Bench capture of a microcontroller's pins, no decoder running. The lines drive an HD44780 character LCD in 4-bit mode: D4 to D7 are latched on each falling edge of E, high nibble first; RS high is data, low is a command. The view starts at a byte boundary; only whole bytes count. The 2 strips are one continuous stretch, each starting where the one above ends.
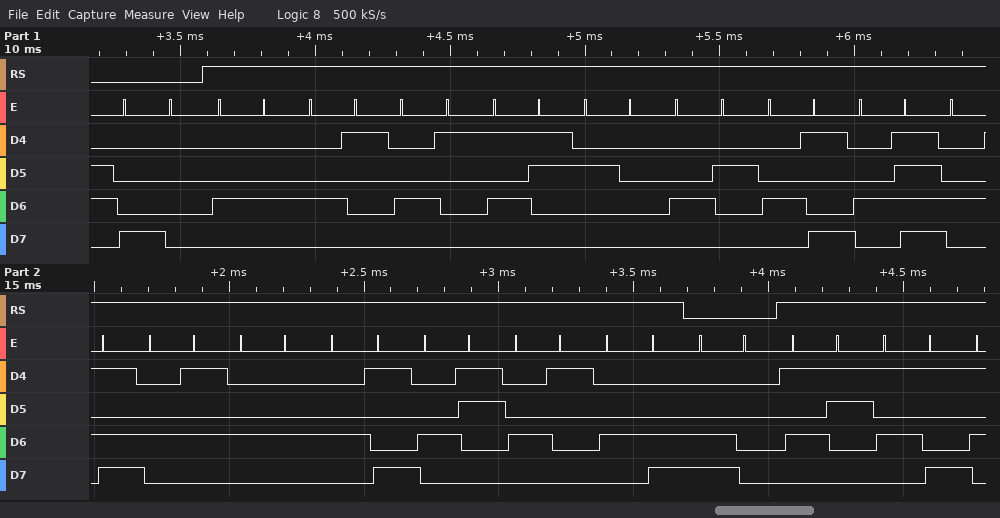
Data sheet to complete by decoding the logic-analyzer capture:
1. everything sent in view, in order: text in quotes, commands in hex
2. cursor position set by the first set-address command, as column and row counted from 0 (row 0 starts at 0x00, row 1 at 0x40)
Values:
0x80 "DAAS BIOMEDICAL" 0xC0 "SY"
column 0, row 0
